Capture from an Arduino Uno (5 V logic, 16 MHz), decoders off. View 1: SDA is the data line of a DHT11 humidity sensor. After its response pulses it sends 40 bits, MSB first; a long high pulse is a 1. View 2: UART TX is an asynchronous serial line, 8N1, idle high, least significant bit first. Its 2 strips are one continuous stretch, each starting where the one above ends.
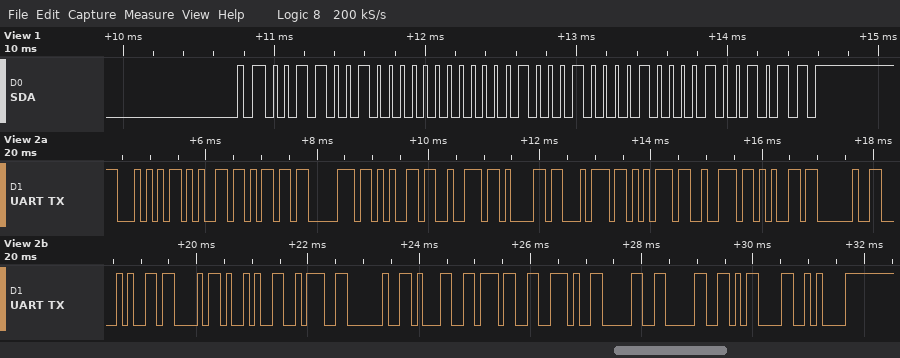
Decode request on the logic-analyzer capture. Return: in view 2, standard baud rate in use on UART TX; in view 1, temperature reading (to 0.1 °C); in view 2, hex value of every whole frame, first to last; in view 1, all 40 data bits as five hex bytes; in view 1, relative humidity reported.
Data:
9600 baud
17.8 °C
54 65 6D 70 65 72 61 74 75 72 65 20 28 43 29 3A 20 31 37 2E 30 30 0D 0A
32 00 11 08 4B
50 %
